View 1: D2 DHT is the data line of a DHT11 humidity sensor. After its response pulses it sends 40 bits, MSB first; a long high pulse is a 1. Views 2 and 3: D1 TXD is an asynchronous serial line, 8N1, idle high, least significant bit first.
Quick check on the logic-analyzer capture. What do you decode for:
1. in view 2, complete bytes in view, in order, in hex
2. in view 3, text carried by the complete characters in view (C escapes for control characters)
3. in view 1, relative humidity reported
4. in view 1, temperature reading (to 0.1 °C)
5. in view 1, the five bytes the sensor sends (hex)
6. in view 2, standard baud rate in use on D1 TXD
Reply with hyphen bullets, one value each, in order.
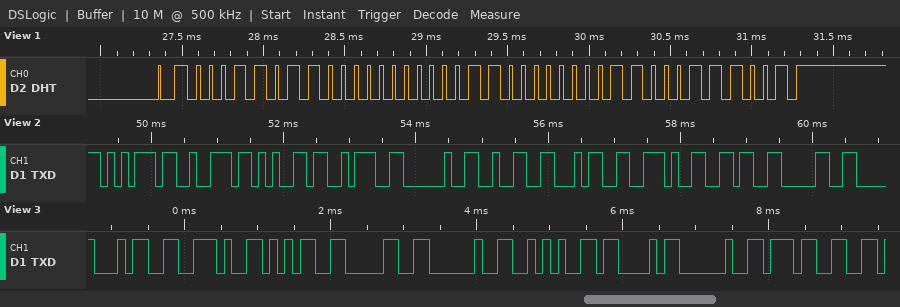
- 75 72 65 3A 20 32 34 2E 36 30
- "4.50 *C 7"
- 27 %
- 24.6 °C
- 1B 00 18 06 39
- 9600 baud
